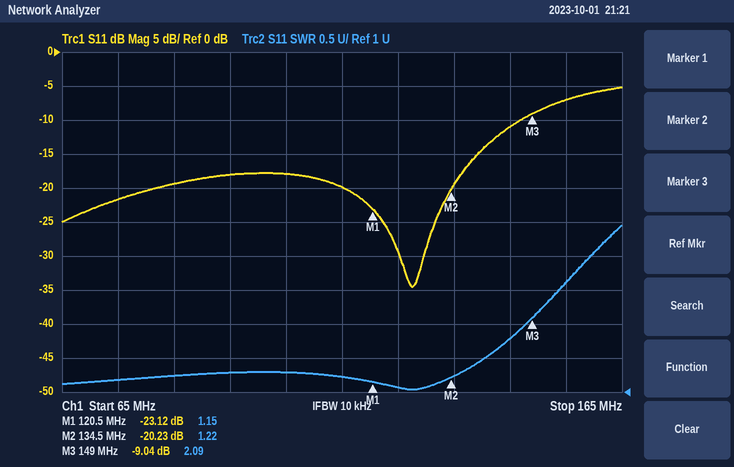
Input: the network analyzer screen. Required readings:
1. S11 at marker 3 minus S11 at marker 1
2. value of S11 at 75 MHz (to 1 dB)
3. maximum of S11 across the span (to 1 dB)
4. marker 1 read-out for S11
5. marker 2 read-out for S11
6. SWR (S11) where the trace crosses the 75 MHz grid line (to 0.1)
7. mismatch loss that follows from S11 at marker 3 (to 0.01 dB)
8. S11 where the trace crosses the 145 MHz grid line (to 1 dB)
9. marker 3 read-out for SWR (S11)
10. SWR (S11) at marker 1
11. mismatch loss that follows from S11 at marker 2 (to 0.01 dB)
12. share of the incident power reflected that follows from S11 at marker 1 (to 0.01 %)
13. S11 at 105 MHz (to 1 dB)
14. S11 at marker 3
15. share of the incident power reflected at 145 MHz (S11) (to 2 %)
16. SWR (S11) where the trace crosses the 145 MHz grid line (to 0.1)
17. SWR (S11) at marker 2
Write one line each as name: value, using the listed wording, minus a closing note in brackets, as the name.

S11 at marker 3 minus S11 at marker 1: 14.08 dB
value of S11 at 75 MHz: -22 dB
maximum of S11 across the span: -5 dB
marker 1 read-out for S11: -23.12 dB
marker 2 read-out for S11: -20.23 dB
SWR (S11) where the trace crosses the 75 MHz grid line: 1.2
mismatch loss that follows from S11 at marker 3: 0.58 dB
S11 where the trace crosses the 145 MHz grid line: -11 dB
marker 3 read-out for SWR: 2.09
SWR (S11) at marker 1: 1.15
mismatch loss that follows from S11 at marker 2: 0.04 dB
share of the incident power reflected that follows from S11 at marker 1: 0.49 %
S11 at 105 MHz: -18 dB
S11 at marker 3: -9.04 dB
share of the incident power reflected at 145 MHz (S11): 8 %
SWR (S11) where the trace crosses the 145 MHz grid line: 1.8
SWR (S11) at marker 2: 1.22
